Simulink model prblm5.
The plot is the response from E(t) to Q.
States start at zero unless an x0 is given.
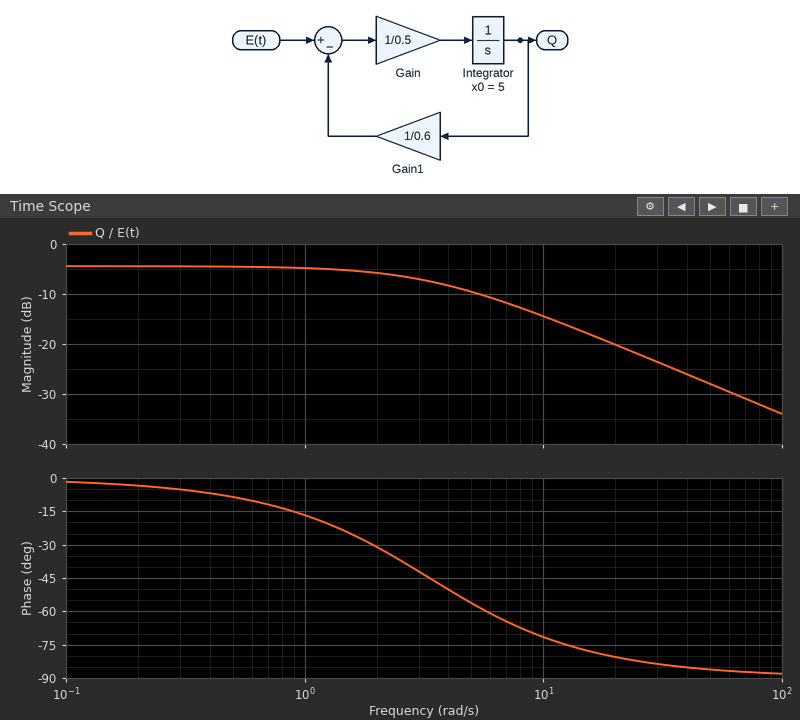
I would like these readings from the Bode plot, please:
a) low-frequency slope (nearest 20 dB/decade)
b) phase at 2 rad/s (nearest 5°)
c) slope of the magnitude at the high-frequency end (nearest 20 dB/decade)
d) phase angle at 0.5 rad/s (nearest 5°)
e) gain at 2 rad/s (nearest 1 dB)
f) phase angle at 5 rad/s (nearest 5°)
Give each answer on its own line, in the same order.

0 dB/decade
-30°
-20 dB/decade
-10°
-6 dB
-55°
